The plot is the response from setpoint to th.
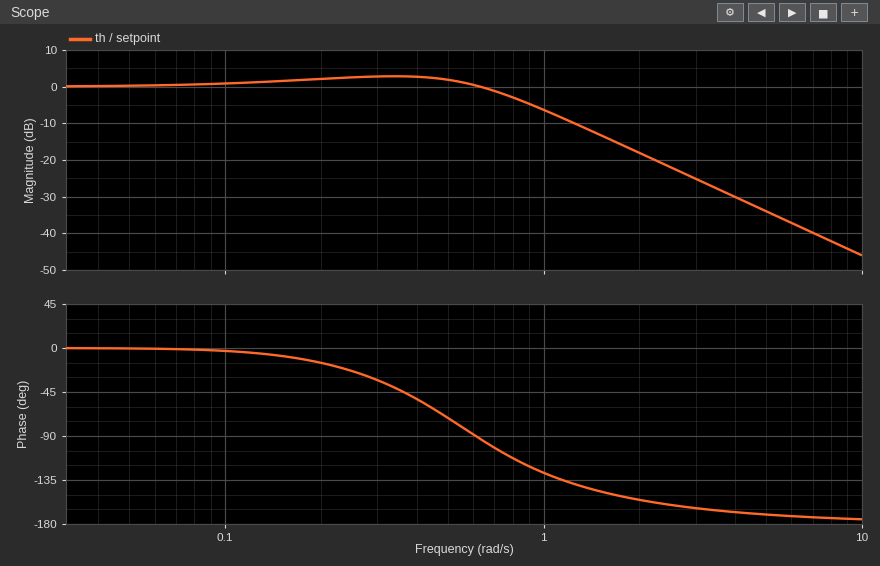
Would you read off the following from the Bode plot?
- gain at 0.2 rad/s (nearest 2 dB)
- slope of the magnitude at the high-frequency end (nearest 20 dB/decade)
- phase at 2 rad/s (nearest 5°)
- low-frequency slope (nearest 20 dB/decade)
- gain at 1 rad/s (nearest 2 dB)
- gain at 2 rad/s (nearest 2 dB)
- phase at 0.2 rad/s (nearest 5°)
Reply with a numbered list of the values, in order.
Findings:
1. 2 dB
2. -40 dB/decade
3. -155°
4. 0 dB/decade
5. -6 dB
6. -18 dB
7. -15°
